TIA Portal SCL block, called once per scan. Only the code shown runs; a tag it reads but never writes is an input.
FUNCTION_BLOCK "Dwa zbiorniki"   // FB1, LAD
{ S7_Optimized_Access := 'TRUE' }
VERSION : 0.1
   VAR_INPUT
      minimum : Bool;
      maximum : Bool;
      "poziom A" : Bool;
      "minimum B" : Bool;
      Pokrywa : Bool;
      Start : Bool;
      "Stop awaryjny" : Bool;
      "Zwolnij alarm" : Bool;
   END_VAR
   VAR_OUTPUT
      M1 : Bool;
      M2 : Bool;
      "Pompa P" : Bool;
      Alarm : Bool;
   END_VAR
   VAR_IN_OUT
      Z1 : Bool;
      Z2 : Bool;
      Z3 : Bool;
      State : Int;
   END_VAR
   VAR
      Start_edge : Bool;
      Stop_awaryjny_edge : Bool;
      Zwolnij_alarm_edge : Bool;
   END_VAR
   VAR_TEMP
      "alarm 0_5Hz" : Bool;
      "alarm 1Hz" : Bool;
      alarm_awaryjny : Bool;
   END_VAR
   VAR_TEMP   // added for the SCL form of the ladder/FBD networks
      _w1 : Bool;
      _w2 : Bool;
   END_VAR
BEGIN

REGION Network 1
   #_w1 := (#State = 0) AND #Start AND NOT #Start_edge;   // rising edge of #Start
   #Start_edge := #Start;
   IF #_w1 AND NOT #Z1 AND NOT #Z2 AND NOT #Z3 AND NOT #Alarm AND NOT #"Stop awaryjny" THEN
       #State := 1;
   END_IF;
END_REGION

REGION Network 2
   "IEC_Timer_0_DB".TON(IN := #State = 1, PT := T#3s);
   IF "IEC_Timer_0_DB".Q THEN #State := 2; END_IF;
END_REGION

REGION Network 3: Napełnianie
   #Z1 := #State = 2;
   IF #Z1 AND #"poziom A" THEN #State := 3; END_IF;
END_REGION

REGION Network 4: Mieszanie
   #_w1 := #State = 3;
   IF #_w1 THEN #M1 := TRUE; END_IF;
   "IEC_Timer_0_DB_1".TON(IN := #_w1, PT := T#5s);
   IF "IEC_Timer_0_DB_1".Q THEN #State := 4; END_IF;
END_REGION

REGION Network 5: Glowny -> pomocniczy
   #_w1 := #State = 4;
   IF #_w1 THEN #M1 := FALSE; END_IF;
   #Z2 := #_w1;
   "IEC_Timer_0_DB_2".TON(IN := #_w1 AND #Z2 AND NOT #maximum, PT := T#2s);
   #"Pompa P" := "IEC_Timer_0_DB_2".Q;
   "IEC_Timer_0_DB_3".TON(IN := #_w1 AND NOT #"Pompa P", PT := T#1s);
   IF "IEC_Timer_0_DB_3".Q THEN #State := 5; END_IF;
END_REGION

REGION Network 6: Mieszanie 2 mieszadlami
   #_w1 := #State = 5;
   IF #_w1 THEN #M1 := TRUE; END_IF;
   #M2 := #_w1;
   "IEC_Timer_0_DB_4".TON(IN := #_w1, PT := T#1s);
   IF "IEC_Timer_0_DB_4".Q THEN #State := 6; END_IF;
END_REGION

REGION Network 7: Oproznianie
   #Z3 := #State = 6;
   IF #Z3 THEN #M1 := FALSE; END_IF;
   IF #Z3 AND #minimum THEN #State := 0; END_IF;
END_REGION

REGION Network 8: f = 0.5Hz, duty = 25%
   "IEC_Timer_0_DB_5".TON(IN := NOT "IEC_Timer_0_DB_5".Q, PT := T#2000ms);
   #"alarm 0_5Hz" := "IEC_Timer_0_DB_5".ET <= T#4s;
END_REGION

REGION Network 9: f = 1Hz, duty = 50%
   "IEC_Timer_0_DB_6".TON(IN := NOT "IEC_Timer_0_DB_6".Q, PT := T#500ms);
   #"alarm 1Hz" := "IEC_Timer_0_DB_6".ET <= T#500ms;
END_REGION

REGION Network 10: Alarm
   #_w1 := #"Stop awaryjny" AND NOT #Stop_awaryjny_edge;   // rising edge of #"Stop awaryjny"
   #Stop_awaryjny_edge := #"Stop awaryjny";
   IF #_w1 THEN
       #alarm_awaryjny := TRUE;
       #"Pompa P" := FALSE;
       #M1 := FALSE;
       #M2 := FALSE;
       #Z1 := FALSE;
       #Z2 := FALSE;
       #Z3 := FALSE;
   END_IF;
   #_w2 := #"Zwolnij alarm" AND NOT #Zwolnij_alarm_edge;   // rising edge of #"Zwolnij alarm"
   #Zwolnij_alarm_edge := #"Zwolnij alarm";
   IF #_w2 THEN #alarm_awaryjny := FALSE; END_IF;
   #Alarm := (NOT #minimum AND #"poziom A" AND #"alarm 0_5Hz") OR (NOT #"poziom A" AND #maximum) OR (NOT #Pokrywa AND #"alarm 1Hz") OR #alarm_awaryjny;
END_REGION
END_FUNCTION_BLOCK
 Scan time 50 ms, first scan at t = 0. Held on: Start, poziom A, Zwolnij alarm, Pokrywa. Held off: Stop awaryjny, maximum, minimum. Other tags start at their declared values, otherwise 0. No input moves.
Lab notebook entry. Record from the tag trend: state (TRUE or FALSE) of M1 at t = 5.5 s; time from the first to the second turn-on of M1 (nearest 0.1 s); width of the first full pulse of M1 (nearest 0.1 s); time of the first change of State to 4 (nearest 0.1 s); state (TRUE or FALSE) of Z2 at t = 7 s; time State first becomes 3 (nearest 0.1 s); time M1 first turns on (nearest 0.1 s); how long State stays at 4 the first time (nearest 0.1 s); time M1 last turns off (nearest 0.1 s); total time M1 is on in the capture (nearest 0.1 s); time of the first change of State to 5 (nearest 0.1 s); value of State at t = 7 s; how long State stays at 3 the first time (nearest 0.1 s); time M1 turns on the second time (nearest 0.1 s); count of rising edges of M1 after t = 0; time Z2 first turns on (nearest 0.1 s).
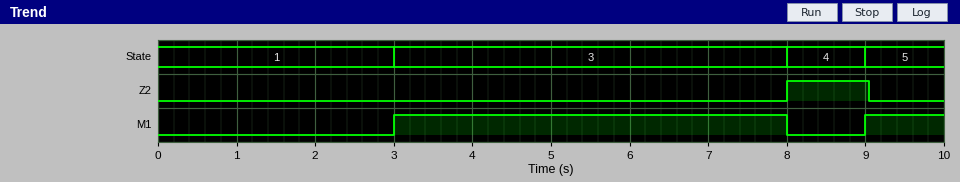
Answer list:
TRUE
6.0 s
5.0 s
8.0 s
FALSE
3.0 s
3.0 s
1.0 s
8.0 s
6.0 s
9.0 s
3
5.0 s
9.0 s
2
8.0 s
